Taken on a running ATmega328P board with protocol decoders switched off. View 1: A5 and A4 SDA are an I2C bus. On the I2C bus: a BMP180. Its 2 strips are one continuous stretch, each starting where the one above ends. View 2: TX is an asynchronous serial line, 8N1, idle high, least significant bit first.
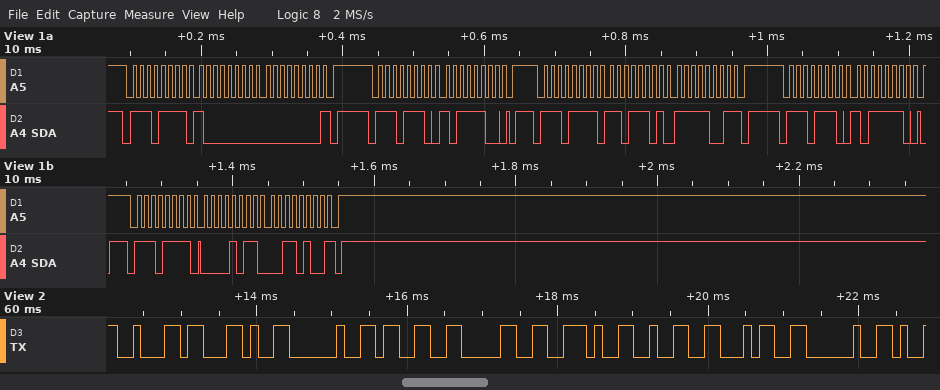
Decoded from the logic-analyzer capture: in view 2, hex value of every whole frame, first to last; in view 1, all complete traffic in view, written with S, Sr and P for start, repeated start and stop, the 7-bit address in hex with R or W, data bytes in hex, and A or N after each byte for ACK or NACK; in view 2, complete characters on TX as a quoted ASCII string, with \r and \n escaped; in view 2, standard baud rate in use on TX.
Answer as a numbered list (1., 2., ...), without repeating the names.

1. 0x62 0x2C 0x20 0x33 0x30 0x2E 0x32 0x34 0x20
2. S 77R A 80 A 00 N P S 77W A BC A P S 77R A DD A F9 N P S 77W A BE A P S 77R A 0B A 34 N P
3. "b, 30.24 "
4. 9600 baud
